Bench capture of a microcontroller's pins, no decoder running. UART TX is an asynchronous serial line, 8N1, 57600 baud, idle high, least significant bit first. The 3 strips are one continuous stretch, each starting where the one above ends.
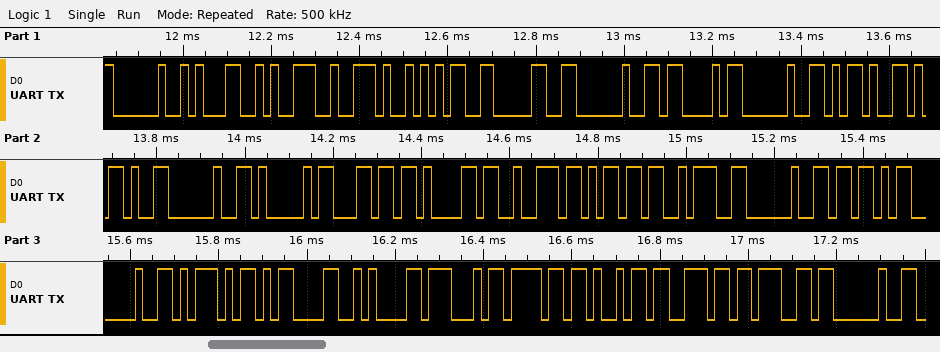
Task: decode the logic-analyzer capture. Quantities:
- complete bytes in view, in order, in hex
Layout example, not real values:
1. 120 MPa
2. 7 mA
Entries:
1. 20 31 39 2E 35 30 20 43 20 2D 2D 20 41 6C 61 72 6D 3A 20 5B 20 5D 0D 0A 47 6F 69 6E 67 20
